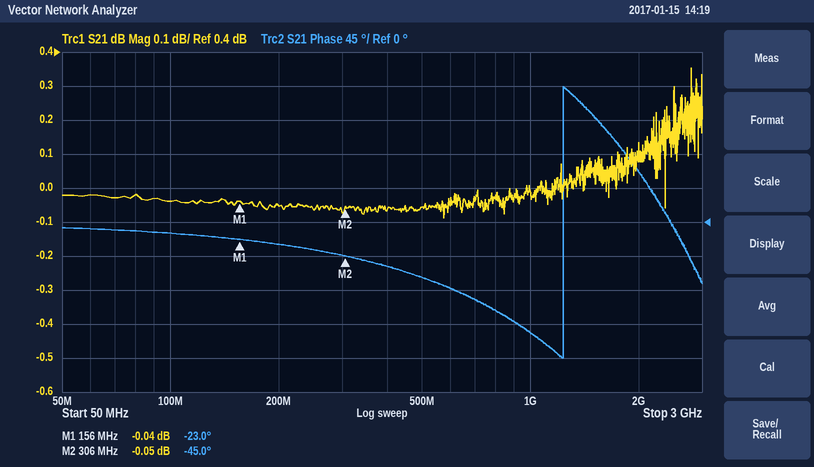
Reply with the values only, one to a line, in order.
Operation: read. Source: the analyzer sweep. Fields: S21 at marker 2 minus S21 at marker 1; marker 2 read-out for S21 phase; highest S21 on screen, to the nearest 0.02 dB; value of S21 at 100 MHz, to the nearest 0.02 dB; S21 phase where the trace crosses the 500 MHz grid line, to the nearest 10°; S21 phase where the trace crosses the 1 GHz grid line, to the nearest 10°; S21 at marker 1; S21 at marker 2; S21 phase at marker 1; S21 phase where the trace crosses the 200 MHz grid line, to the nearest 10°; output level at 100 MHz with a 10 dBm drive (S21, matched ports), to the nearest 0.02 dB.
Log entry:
-0.01 dB
-45.0°
0.36 dB
-0.04 dB
-70°
-150°
-0.04 dB
-0.05 dB
-23.0°
-30°
9.96 dBm
